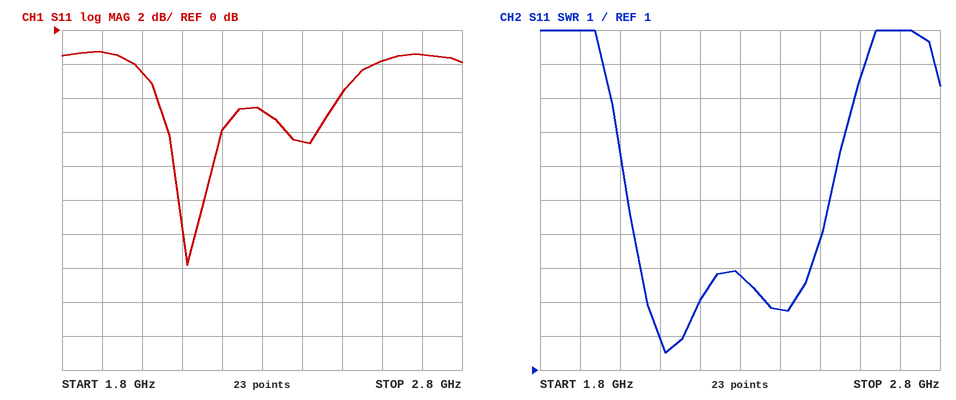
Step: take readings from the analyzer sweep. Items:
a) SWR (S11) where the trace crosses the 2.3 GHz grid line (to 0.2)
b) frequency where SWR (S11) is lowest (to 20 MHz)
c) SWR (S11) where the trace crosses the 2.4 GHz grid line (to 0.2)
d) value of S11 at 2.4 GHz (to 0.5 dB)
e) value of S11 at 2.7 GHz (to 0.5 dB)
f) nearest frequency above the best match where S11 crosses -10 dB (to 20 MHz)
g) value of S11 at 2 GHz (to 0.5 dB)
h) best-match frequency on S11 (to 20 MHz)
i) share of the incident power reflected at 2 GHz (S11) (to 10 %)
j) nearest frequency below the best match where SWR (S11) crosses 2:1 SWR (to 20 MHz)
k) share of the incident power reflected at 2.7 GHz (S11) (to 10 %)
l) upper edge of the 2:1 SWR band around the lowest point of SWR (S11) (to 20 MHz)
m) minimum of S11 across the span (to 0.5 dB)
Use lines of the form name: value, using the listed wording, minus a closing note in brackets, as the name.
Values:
SWR (S11) where the trace crosses the 2.3 GHz grid line: 3.8
frequency where SWR (S11) is lowest: 2.12 GHz
SWR (S11) where the trace crosses the 2.4 GHz grid line: 2.8
value of S11 at 2.4 GHz: -6.5 dB
value of S11 at 2.7 GHz: -1.5 dB
nearest frequency above the best match where S11 crosses -10 dB: 2.16 GHz
value of S11 at 2 GHz: -2.5 dB
best-match frequency on S11: 2.12 GHz
share of the incident power reflected at 2 GHz (S11): 60 %
nearest frequency below the best match where SWR (S11) crosses 2:1 SWR: 2.10 GHz
share of the incident power reflected at 2.7 GHz (S11): 70 %
upper edge of the 2:1 SWR band around the lowest point of SWR (S11): 2.16 GHz
minimum of S11 across the span: -14.0 dB
